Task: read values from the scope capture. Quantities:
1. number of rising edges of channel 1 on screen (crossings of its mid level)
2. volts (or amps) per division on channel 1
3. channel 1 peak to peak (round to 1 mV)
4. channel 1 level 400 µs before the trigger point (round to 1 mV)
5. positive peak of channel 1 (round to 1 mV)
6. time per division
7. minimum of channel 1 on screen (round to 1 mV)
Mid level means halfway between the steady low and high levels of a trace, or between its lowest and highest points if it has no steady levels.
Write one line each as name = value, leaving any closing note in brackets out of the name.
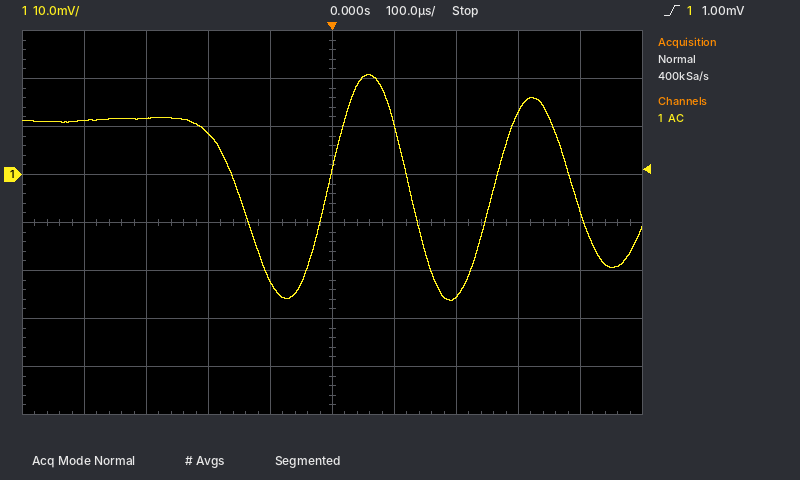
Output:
number of rising edges of channel 1 on screen = 2
volts (or amps) per division on channel 1 = 10 mV
channel 1 peak to peak = 47 mV
channel 1 level 400 µs before the trigger point = 11 mV
positive peak of channel 1 = 21 mV
time per division = 100 µs
minimum of channel 1 on screen = -26 mV
